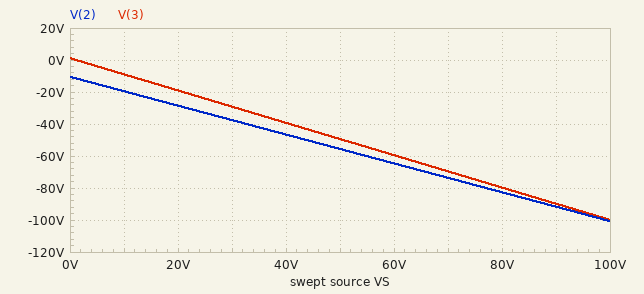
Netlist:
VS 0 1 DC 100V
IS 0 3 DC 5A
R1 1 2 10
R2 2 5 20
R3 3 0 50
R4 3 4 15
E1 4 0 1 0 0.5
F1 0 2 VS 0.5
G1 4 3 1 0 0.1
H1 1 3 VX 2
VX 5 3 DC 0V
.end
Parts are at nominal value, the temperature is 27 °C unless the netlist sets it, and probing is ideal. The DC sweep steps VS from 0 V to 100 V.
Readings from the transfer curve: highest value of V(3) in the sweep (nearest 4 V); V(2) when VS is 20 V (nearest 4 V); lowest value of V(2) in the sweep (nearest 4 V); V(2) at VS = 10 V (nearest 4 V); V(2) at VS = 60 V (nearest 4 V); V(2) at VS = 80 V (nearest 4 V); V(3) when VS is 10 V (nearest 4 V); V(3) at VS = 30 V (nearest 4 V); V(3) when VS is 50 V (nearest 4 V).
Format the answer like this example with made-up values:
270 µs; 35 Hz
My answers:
0 V; -28 V; -100 V; -20 V; -64 V; -84 V; -8 V; -28 V; -48 V
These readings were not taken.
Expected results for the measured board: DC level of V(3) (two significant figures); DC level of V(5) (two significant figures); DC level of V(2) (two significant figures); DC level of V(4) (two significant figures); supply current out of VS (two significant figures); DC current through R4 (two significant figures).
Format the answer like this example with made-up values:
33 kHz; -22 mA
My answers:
-100 V; -100 V; -100 V; -50 V; 220 mA; 3.3 A
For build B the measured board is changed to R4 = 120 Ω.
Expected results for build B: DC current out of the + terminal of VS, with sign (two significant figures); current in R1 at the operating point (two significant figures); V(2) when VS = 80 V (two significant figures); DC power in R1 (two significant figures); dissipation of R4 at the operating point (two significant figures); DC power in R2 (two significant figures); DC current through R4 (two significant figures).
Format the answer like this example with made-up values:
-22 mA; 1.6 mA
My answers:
-1.7 A; 550 mA; -78 V; 3.0 W; 21 W; 1.9 W; 420 mA
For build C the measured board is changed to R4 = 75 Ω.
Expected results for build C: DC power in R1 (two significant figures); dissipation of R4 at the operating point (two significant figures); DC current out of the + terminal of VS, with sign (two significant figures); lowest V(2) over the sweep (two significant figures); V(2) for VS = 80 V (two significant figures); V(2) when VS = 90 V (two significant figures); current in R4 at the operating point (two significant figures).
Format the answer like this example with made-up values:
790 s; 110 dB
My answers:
2.5 W; 34 W; -1.5 A; -95 V; -78 V; -87 V; 670 mA
